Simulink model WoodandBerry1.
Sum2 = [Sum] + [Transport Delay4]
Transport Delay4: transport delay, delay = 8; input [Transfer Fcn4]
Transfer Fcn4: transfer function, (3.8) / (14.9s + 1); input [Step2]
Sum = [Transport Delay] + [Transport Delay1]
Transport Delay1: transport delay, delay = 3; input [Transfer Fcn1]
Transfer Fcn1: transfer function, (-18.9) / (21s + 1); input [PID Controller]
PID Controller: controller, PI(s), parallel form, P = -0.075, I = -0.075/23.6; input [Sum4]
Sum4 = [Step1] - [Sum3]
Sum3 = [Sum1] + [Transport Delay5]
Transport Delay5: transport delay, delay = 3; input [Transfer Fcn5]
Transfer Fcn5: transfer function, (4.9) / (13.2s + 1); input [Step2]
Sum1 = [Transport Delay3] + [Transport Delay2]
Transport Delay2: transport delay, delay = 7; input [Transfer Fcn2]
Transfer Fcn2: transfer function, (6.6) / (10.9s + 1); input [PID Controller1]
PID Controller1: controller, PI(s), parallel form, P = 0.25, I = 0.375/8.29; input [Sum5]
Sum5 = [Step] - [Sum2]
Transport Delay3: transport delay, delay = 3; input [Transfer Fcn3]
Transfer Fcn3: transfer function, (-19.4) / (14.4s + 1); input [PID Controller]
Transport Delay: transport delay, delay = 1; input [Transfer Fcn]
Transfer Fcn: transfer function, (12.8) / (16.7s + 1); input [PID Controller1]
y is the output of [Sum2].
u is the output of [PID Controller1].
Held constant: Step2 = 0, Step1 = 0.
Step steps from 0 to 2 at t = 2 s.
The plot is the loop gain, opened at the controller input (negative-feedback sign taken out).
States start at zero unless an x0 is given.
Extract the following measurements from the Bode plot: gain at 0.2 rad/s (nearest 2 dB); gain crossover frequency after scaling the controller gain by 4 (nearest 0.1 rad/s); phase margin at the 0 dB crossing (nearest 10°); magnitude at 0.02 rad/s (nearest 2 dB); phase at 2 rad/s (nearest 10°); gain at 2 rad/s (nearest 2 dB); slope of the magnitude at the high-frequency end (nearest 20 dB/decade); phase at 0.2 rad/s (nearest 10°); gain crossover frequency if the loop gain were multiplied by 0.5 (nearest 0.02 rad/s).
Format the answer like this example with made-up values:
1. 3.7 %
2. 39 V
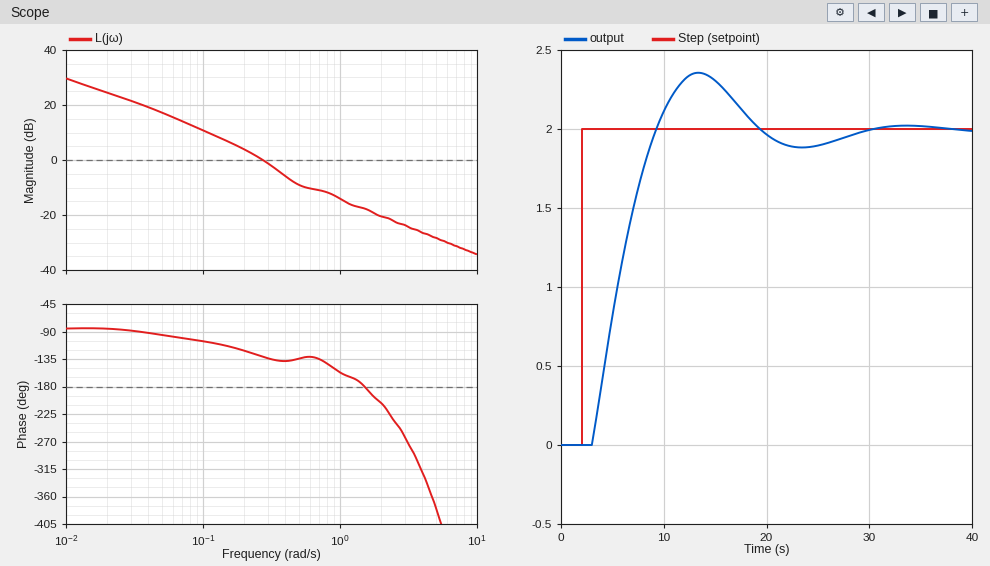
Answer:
1. 4 dB
2. 0.8 rad/s
3. 50°
4. 24 dB
5. -210°
6. -20 dB
7. -20 dB/decade
8. -120°
9. 0.16 rad/s
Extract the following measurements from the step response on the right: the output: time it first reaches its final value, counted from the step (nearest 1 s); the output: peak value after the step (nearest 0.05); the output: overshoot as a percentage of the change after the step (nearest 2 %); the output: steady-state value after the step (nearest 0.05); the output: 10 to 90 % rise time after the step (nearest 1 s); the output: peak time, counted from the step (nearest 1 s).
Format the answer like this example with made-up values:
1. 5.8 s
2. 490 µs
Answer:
1. 7 s
2. 2.35
3. 18 %
4. 2.00
5. 5 s
6. 11 s
